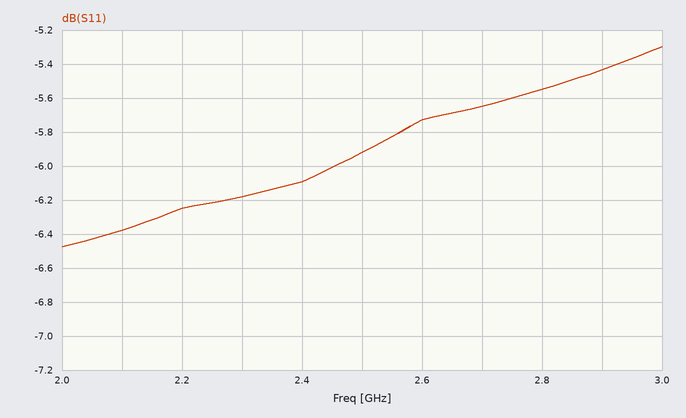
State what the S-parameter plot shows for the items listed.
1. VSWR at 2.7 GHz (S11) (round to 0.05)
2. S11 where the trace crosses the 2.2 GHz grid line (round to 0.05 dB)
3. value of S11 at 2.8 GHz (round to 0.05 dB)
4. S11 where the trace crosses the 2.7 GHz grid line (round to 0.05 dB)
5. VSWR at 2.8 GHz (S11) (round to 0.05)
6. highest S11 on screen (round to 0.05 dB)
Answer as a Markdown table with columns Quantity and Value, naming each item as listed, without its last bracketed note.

| Quantity | Value |
|---|---|
| VSWR at 2.7 GHz (S11) | 3.20 |
| S11 where the trace crosses the 2.2 GHz grid line | -6.25 dB |
| value of S11 at 2.8 GHz | -5.55 dB |
| S11 where the trace crosses the 2.7 GHz grid line | -5.65 dB |
| VSWR at 2.8 GHz (S11) | 3.25 |
| highest S11 on screen | -5.30 dB |
